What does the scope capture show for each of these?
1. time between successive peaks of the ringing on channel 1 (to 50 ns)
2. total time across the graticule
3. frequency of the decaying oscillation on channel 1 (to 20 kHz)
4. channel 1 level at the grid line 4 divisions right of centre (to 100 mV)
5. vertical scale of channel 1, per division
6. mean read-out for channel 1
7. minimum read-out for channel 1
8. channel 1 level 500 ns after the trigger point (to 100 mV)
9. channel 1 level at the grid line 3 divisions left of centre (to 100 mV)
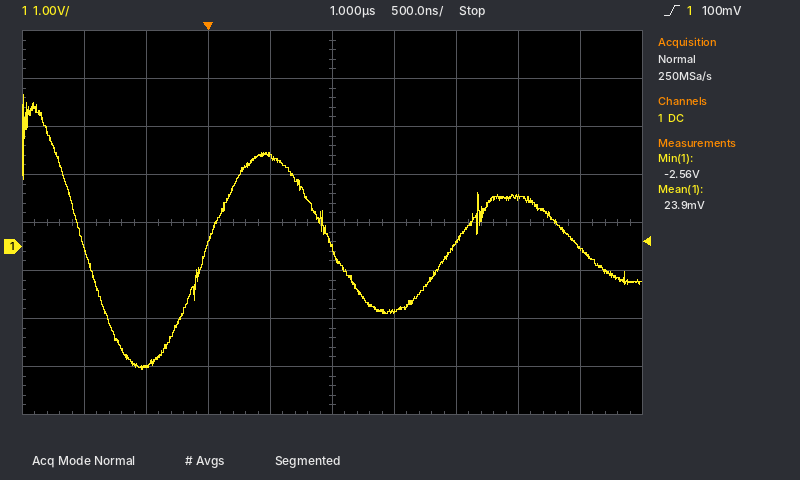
1.95 µs
5 µs
520 kHz
0.0 V
1 V
23.9 mV
-2.56 V
1.9 V
-2.5 V
